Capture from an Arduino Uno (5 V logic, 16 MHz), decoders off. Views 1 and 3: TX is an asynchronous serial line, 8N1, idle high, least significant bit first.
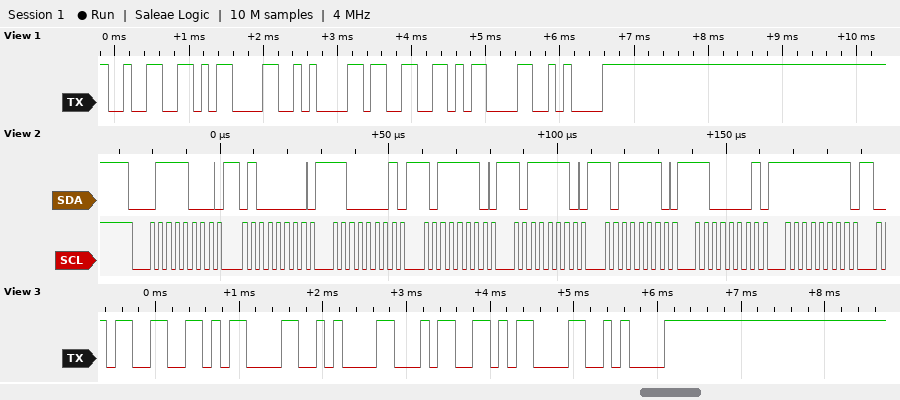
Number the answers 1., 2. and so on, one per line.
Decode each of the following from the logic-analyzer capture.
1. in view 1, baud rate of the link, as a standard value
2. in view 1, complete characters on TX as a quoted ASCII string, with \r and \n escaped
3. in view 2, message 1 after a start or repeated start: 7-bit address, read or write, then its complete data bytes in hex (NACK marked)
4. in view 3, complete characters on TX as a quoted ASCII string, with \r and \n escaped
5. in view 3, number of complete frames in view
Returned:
1. 9600 baud
2. "2\r\n3\r\n"
3. 0x3C write: 40 C1 BE BE BE C1 FF
4. "3\r\n4\r\n"
5. 6
